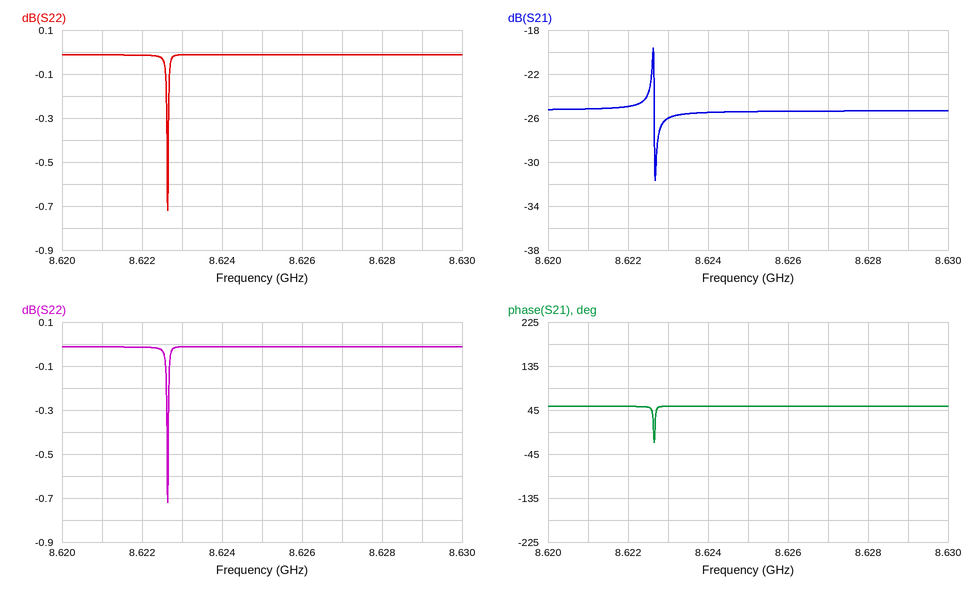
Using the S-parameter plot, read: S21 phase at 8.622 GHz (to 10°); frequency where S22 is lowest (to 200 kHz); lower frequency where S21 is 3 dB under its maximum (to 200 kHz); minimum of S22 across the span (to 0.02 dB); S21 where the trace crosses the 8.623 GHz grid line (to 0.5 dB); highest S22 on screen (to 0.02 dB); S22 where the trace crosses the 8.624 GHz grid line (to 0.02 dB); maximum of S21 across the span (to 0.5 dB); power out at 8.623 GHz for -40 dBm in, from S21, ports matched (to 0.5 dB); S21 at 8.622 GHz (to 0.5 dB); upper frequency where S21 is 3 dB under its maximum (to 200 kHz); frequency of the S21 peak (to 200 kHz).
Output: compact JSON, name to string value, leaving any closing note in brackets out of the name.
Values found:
{"S21 phase at 8.622 GHz": "50°", "frequency where S22 is lowest": "8.6226 GHz", "lower frequency where S21 is 3 dB under its maximum": "8.6226 GHz", "minimum of S22 across the span": "-0.72 dB", "S21 where the trace crosses the 8.623 GHz grid line": "-26.0 dB", "highest S22 on screen": "-0.02 dB", "S22 where the trace crosses the 8.624 GHz grid line": "-0.02 dB", "maximum of S21 across the span": "-19.5 dB", "power out at 8.623 GHz for -40 dBm in, from S21, ports matched": "-66.0 dBm", "S21 at 8.622 GHz": "-25.0 dB", "upper frequency where S21 is 3 dB under its maximum": "8.6226 GHz", "frequency of the S21 peak": "8.6226 GHz"}
